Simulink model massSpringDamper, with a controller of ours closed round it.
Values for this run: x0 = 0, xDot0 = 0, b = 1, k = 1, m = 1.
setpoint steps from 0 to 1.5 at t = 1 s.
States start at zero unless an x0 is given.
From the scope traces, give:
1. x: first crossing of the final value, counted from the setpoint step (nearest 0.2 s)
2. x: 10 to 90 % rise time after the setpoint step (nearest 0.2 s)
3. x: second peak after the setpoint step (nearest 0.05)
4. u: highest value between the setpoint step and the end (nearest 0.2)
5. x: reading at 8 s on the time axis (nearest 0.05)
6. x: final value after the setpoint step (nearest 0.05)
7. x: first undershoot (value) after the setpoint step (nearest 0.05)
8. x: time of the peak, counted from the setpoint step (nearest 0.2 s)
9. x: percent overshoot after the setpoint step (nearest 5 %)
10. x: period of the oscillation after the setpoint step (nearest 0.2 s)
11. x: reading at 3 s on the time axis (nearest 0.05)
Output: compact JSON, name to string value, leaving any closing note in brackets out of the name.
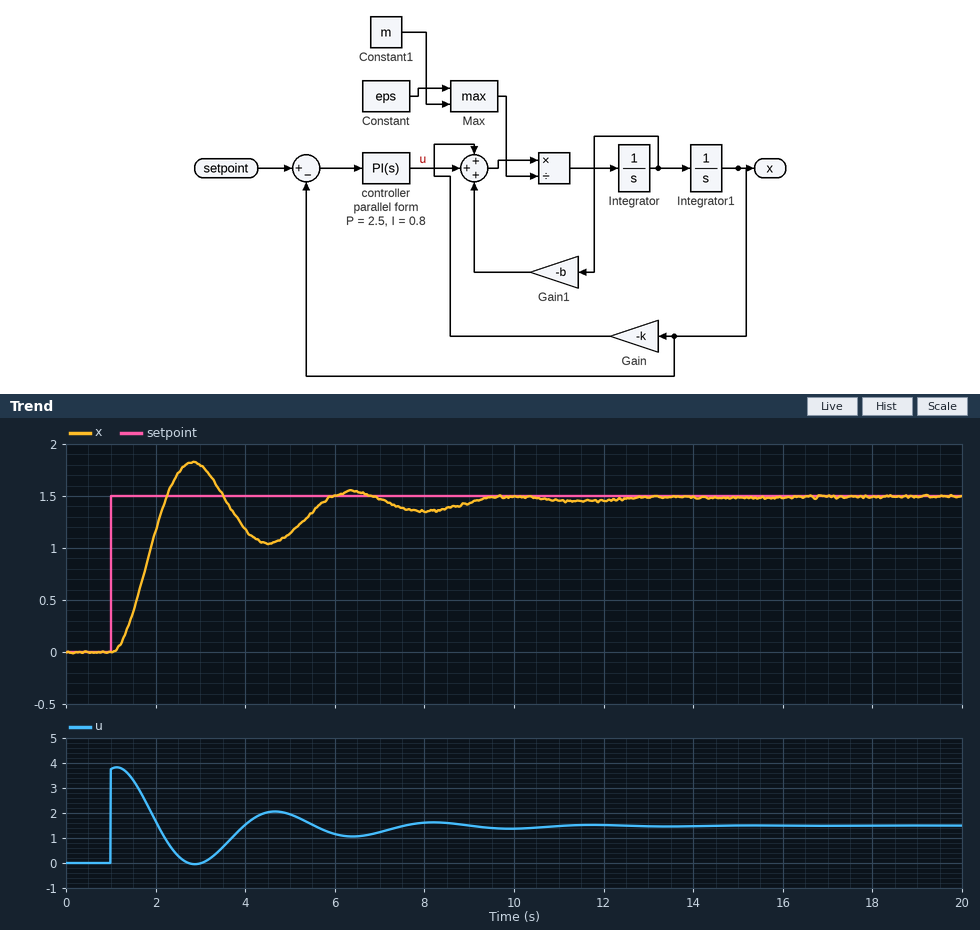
{"x: first crossing of the final value, counted from the setpoint step": "1.2 s", "x: 10 to 90 % rise time after the setpoint step": "0.8 s", "x: second peak after the setpoint step": "1.55", "u: highest value between the setpoint step and the end": "3.8", "x: reading at 8 s on the time axis": "1.35", "x: final value after the setpoint step": "1.50", "x: first undershoot (value) after the setpoint step": "1.05", "x: time of the peak, counted from the setpoint step": "1.8 s", "x: percent overshoot after the setpoint step": "20 %", "x: period of the oscillation after the setpoint step": "3.6 s", "x: reading at 3 s on the time axis": "1.80"}
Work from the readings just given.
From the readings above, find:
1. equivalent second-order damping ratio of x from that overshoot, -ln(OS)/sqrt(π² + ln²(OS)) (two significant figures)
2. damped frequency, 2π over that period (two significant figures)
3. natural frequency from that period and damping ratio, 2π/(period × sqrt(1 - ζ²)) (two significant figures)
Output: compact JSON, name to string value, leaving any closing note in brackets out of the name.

{"equivalent second-order damping ratio of x from that overshoot, -ln(OS)/sqrt(π² + ln²(OS))": "0.46", "damped frequency, 2π over that period": "1.7 rad/s", "natural frequency from that period and damping ratio, 2π/(period × sqrt(1 - ζ²))": "2.0 rad/s"}
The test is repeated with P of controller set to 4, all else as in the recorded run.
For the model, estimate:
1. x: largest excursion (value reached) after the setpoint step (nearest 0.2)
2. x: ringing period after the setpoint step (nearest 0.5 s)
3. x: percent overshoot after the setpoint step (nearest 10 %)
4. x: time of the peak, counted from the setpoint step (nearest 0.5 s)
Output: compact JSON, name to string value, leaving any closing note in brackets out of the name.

{"x: largest excursion (value reached) after the setpoint step": "2.0", "x: ringing period after the setpoint step": "3.0 s", "x: percent overshoot after the setpoint step": "30 %", "x: time of the peak, counted from the setpoint step": "1.5 s"}
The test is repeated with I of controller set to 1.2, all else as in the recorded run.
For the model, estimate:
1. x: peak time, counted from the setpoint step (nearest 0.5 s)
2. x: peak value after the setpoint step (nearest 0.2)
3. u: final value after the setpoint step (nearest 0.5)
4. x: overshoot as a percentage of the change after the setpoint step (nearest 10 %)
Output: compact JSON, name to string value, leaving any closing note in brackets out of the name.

{"x: peak time, counted from the setpoint step": "2.0 s", "x: peak value after the setpoint step": "2.0", "u: final value after the setpoint step": "1.5", "x: overshoot as a percentage of the change after the setpoint step": "30 %"}
